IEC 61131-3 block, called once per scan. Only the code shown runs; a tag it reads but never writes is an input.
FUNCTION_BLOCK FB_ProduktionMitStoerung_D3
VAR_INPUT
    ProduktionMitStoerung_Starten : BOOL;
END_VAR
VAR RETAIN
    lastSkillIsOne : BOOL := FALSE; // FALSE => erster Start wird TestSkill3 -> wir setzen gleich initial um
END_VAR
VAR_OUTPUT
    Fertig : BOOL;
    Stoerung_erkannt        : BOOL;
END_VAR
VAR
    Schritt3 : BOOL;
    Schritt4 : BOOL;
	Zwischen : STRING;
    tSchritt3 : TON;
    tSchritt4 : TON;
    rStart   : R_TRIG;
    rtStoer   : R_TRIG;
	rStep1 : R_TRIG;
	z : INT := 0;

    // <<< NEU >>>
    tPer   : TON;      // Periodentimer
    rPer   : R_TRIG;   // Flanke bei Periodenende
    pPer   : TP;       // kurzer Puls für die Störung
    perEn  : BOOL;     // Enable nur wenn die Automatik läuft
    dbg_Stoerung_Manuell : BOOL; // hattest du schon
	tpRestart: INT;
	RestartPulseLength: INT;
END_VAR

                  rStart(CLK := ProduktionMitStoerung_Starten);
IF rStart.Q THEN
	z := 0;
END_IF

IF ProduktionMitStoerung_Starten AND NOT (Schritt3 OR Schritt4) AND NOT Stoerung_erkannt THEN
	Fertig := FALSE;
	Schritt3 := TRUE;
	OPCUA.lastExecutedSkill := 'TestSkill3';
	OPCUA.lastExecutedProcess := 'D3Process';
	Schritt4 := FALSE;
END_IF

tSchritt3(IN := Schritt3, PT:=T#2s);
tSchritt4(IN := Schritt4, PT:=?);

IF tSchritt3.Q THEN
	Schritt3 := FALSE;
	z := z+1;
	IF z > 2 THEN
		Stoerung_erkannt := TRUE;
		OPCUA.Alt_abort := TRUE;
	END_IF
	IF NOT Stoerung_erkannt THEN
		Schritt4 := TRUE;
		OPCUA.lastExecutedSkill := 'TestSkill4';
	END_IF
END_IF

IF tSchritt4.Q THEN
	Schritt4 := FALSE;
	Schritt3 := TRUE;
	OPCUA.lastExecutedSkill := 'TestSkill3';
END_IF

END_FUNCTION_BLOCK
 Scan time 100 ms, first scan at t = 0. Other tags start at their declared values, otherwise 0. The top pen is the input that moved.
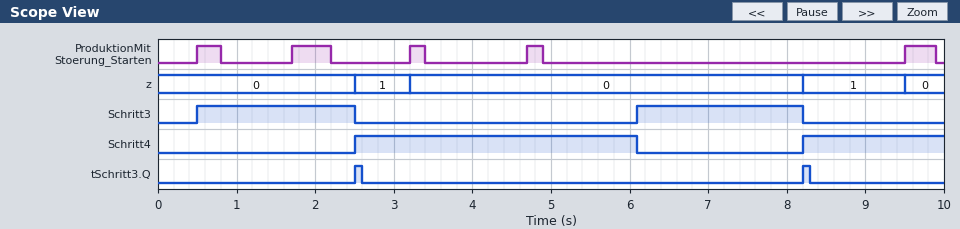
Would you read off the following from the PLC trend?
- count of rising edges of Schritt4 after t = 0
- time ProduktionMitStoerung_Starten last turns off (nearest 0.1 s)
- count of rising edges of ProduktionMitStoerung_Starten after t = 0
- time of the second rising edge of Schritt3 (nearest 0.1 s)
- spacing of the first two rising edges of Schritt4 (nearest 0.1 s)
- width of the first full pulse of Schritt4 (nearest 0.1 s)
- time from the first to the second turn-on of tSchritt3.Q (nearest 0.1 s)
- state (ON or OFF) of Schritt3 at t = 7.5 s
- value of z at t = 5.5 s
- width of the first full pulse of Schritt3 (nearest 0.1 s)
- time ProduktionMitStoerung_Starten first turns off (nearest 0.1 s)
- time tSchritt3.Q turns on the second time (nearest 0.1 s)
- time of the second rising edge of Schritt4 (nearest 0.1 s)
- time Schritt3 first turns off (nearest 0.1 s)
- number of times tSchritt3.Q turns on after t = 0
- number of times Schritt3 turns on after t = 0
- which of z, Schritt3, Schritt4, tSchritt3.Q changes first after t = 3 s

2
9.9 s
5
6.1 s
5.7 s
3.6 s
5.7 s
ON
0
2.0 s
0.8 s
8.2 s
8.2 s
2.5 s
2
2
z
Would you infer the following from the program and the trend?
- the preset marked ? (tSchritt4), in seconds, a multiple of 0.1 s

3.5 s
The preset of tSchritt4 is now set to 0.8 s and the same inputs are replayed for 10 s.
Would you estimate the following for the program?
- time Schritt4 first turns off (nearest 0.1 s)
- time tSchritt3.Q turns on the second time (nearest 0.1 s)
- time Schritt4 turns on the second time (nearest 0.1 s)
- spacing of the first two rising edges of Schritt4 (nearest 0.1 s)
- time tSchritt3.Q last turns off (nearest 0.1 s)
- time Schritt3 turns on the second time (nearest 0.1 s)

3.4 s
5.5 s
5.5 s
3.0 s
8.6 s
3.4 s
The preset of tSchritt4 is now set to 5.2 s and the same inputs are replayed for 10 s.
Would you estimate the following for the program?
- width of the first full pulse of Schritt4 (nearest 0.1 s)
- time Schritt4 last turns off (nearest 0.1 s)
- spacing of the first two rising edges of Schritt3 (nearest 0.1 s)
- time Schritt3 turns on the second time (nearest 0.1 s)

5.3 s
7.8 s
7.3 s
7.8 s
